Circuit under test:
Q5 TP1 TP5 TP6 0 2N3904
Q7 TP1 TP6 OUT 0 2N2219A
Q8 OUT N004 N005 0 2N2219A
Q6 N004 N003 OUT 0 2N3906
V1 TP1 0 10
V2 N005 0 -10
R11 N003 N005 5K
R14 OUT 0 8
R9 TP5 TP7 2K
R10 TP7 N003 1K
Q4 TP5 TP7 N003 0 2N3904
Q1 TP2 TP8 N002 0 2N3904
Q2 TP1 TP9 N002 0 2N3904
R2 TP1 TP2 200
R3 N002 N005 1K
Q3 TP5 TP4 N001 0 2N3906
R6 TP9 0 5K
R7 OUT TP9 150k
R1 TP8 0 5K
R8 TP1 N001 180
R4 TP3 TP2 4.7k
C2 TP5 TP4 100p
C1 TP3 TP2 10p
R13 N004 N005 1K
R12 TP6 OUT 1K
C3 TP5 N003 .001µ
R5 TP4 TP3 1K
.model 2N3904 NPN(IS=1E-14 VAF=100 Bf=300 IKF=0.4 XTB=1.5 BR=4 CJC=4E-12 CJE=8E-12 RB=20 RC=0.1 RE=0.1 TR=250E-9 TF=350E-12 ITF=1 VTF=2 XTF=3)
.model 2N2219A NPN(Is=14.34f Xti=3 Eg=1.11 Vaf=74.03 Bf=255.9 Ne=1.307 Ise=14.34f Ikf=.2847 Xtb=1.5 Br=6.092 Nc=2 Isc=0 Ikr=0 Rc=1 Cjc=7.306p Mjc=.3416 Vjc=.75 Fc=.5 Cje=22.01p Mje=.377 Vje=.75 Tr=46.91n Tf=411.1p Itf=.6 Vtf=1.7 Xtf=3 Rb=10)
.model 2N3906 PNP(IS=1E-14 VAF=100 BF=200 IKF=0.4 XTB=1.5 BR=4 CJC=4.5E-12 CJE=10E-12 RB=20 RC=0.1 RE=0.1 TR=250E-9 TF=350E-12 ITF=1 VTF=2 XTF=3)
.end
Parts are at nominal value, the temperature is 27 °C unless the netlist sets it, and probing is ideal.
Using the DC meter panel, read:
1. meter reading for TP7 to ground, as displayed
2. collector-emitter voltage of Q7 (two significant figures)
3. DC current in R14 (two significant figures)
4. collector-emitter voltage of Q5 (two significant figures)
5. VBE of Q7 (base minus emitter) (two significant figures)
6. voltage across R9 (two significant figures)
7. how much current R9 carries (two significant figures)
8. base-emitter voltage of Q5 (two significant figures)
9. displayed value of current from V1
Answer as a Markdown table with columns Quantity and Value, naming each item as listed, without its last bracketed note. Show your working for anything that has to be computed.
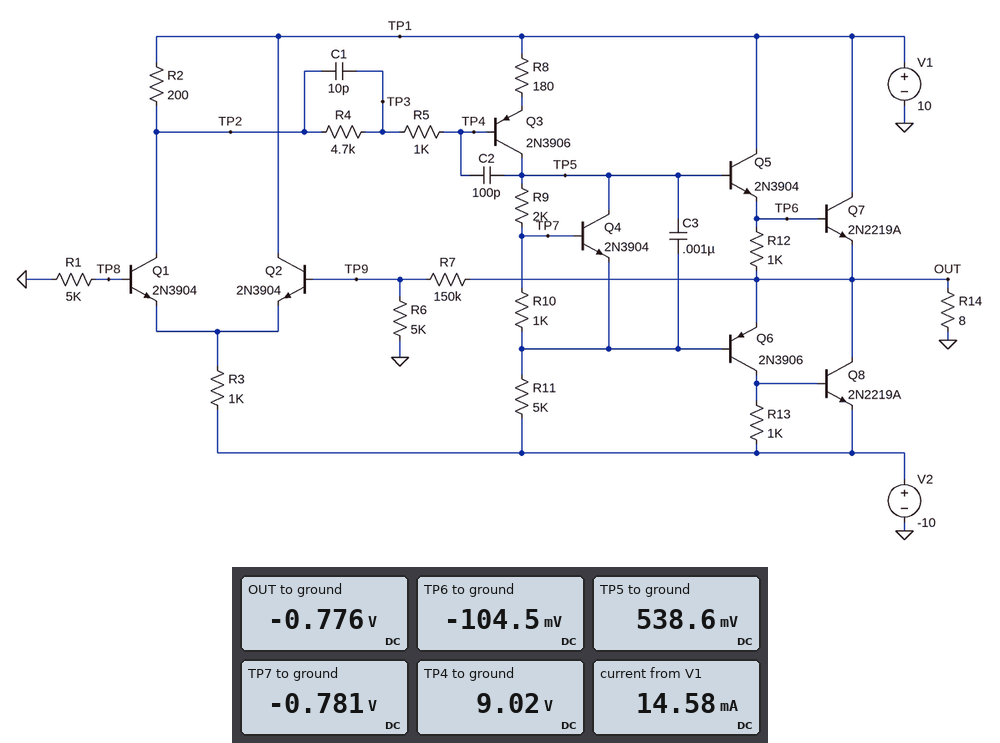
| Quantity | Value |
|---|---|
| meter reading for TP7 to ground, as displayed | -0.781 V |
| collector-emitter voltage of Q7 | 10 V - (-776 mV) = 11 V |
| DC current in R14 | (0 V - (-776 mV)) / 8 Ω = 97 mA |
| collector-emitter voltage of Q5 | 10 V - (-104.5 mV) = 10 V |
| VBE of Q7 (base minus emitter) | -104.5 mV - (-776 mV) = 670 mV |
| voltage across R9 | 538.6 mV - (-781 mV) = 1.3 V |
| how much current R9 carries | (538.6 mV - (-781 mV)) / 2 kΩ = 660 µA |
| base-emitter voltage of Q5 | 538.6 mV - (-104.5 mV) = 640 mV |
| displayed value of current from V1 | 14.58 mA |
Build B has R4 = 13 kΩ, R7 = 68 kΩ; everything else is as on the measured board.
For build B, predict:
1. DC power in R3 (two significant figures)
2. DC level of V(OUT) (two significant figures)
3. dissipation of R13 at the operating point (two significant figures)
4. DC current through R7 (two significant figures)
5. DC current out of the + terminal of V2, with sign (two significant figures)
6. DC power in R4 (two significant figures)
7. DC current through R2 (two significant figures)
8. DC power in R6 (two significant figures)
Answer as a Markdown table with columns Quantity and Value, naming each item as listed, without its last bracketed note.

| Quantity | Value |
|---|---|
| DC power in R3 | 85 mW |
| DC level of V(OUT) | -630 mV |
| dissipation of R13 at the operating point | 590 µW |
| DC current through R7 | 7.8 µA |
| DC current out of the + terminal of V2, with sign | -94 mA |
| DC power in R4 | 840 nW |
| DC current through R2 | 5.5 mA |
| DC power in R6 | 1.8 µW |
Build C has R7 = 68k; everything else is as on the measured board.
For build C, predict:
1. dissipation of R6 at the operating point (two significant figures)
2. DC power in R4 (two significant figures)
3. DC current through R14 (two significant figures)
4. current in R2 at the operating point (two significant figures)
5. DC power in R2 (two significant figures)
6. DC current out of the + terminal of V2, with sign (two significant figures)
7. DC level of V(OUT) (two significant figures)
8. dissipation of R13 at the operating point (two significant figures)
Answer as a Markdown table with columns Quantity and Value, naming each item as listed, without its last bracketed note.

| Quantity | Value |
|---|---|
| dissipation of R6 at the operating point | 1.5 µW |
| DC power in R4 | 320 nW |
| DC current through R14 | 56 mA |
| current in R2 at the operating point | 5.2 mA |
| DC power in R2 | 5.4 mW |
| DC current out of the + terminal of V2, with sign | -72 mA |
| DC level of V(OUT) | -450 mV |
| dissipation of R13 at the operating point | 570 µW |
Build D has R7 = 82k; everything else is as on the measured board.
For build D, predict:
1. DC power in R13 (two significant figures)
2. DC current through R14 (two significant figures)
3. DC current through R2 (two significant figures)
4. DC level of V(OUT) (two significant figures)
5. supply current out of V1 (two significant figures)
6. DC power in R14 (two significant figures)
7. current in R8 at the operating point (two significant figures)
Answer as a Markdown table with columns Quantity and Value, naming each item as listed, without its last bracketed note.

| Quantity | Value |
|---|---|
| DC power in R13 | 580 µW |
| DC current through R14 | 64 mA |
| DC current through R2 | 5.2 mA |
| DC level of V(OUT) | -510 mV |
| supply current out of V1 | 16 mA |
| DC power in R14 | 32 mW |
| current in R8 at the operating point | 1.8 mA |
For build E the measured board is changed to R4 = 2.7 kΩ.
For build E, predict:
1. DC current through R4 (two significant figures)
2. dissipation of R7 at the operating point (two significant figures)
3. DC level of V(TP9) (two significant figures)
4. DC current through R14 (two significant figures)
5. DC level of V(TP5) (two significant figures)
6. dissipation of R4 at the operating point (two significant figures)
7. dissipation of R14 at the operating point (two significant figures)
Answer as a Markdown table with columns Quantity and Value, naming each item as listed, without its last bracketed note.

| Quantity | Value |
|---|---|
| DC current through R4 | 8.0 µA |
| dissipation of R7 at the operating point | 2.5 µW |
| DC level of V(TP9) | -84 mV |
| DC current through R14 | 87 mA |
| DC level of V(TP5) | 620 mV |
| dissipation of R4 at the operating point | 170 nW |
| dissipation of R14 at the operating point | 60 mW |
